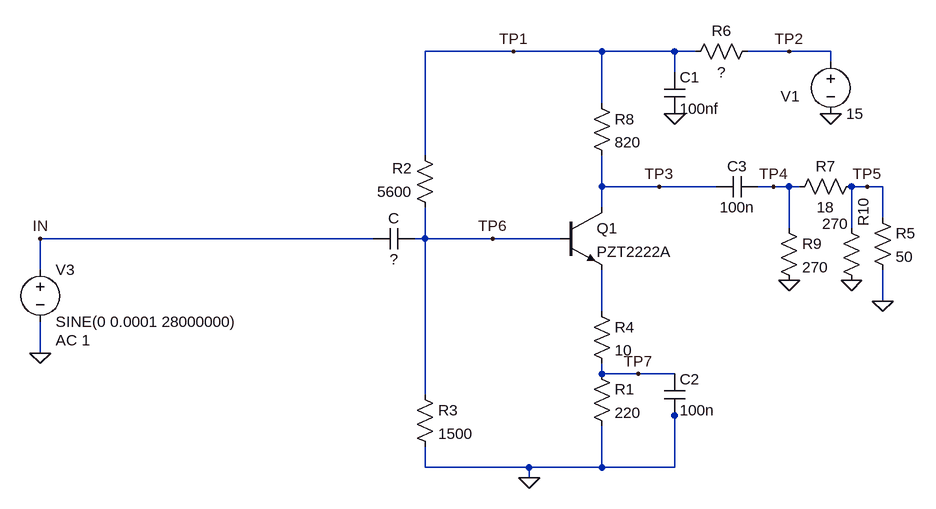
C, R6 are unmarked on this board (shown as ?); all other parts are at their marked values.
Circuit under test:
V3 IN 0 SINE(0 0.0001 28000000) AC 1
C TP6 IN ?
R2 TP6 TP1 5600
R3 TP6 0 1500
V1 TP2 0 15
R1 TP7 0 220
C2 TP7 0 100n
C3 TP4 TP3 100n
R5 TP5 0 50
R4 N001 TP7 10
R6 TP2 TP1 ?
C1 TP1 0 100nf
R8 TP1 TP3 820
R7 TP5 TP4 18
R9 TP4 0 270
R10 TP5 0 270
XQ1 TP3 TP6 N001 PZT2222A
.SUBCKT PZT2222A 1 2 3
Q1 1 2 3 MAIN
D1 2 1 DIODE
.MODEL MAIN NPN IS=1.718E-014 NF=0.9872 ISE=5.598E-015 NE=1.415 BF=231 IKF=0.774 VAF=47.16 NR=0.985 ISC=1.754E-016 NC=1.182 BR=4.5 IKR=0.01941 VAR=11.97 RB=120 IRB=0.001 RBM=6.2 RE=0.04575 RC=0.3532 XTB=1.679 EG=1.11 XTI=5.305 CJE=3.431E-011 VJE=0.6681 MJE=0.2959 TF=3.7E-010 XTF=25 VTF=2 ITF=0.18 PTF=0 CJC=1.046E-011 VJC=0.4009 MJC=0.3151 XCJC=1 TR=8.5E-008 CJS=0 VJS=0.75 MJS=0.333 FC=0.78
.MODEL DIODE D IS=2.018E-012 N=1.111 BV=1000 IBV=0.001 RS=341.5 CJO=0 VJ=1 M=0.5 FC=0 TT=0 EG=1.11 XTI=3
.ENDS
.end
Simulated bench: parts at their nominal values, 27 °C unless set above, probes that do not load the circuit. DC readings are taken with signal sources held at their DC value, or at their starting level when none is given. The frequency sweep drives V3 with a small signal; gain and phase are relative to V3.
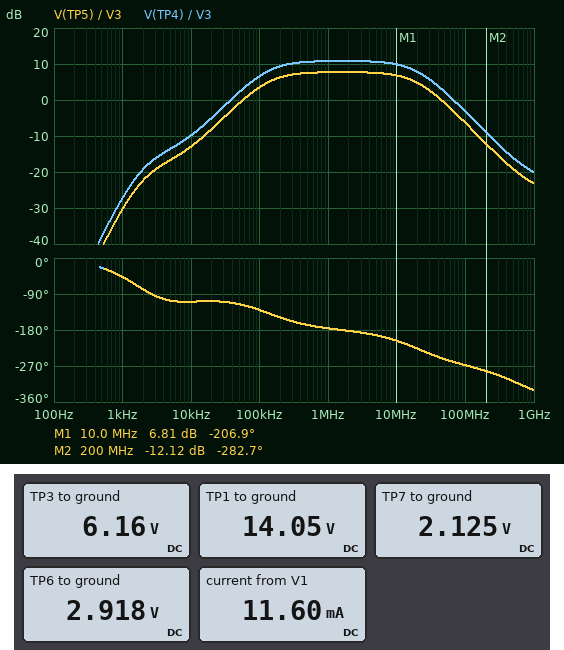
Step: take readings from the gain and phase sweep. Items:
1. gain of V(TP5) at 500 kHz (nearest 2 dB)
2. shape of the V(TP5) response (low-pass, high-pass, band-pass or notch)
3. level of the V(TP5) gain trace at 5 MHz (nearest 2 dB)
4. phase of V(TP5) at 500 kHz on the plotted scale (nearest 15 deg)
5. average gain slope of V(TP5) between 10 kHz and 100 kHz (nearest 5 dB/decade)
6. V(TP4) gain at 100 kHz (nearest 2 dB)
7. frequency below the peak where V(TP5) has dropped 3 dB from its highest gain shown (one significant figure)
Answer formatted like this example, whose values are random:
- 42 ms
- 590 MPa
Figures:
- 8 dB
- band-pass
- 8 dB
- -165 deg
- 15 dB/decade
- 6 dB
- 100 kHz
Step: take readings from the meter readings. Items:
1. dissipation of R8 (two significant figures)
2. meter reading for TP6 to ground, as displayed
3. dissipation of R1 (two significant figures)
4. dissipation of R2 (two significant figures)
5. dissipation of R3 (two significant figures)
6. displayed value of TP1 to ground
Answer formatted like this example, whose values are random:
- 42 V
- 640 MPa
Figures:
- 76 mW
- 2.918 V
- 21 mW
- 22 mW
- 5.7 mW
- 14.05 V
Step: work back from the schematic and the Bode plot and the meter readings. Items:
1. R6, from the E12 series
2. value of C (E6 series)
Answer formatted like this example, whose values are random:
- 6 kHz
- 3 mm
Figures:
- 82 Ω
- 68 nF
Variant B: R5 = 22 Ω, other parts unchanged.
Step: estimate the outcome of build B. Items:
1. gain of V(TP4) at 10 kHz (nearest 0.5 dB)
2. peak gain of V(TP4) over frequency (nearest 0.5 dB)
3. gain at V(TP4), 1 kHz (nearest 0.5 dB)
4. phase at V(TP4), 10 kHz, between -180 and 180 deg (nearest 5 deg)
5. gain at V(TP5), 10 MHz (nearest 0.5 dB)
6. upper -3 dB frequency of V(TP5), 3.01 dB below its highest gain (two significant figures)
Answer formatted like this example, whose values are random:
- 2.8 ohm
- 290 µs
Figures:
- -13.0 dB
- 7.5 dB
- -30.5 dB
- -110 deg
- 1.5 dB
- 22 MHz
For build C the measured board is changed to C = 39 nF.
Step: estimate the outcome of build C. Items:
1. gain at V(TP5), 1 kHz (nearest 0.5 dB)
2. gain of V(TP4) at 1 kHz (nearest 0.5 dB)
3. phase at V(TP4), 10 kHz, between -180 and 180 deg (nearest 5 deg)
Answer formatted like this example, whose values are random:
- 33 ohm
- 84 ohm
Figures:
- -34.5 dB
- -31.5 dB
- -100 deg
